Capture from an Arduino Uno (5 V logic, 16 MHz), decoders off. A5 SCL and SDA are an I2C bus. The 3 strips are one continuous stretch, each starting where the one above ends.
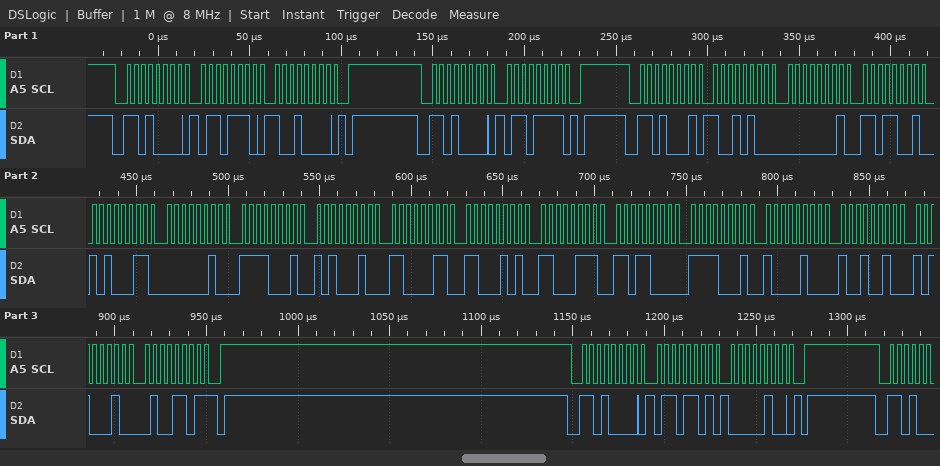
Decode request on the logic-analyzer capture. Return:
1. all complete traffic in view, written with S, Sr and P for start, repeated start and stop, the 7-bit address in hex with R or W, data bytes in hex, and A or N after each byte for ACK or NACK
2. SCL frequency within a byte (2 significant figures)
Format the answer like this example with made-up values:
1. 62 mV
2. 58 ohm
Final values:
1. S 68W A 6E A 90 A P S 68W A 6F A P S 68R A 94 A 01 A D9 A A3 A 02 A F1 A A2 A C3 A C5 A C7 A D8 A F1 A 84 A 92 A A2 A 4D N P S 68W A 6D A 04 A P
2. 250 kHz
